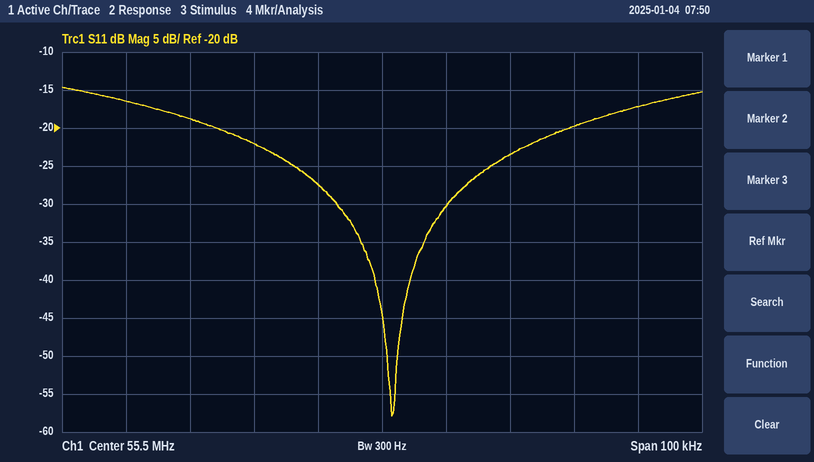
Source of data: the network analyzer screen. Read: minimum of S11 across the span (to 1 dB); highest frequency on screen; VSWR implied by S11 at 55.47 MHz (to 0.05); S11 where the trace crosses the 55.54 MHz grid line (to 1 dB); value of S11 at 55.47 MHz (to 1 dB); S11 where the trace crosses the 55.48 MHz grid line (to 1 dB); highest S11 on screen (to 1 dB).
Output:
-58 dB
55.55 MHz
1.25
-17 dB
-19 dB
-22 dB
-15 dB
